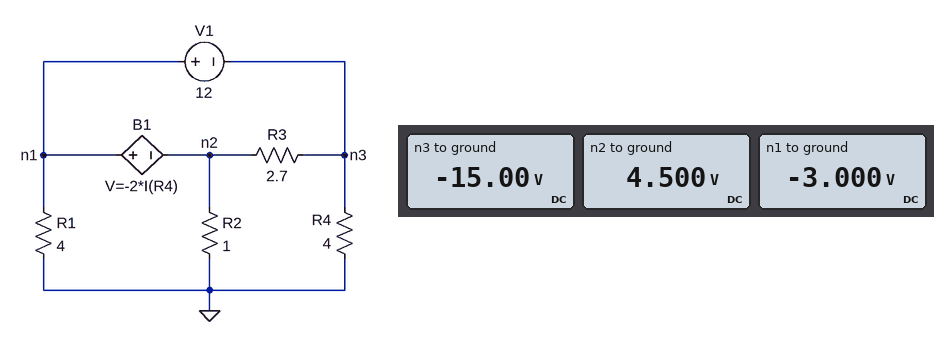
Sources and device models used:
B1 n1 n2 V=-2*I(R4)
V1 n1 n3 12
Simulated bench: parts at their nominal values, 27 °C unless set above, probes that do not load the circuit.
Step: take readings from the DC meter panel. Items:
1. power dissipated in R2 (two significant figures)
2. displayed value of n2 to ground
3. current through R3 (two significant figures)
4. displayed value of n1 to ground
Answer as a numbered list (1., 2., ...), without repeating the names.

1. 20 W
2. 4.500 V
3. 7.2 A
4. -3.000 V
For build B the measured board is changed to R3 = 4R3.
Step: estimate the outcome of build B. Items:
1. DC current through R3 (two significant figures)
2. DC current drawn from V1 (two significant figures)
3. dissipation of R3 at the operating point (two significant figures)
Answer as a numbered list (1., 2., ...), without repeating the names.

1. 4.5 A
2. 8.3 A
3. 88 W
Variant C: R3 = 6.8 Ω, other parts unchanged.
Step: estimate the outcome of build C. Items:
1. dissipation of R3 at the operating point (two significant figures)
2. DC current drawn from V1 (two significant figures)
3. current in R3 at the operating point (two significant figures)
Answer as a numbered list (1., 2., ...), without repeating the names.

1. 56 W
2. 6.6 A
3. 2.9 A
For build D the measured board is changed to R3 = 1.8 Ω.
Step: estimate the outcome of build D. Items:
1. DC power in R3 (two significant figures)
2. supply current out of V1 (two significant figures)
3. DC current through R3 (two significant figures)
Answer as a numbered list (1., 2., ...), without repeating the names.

1. 210 W
2. 15 A
3. 11 A
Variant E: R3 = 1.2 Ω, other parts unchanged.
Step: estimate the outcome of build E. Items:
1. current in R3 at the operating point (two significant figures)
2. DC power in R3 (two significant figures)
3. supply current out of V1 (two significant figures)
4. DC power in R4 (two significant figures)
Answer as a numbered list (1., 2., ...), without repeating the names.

1. 16 A
2. 320 W
3. 20 A
4. 56 W
